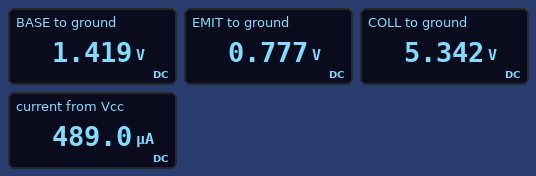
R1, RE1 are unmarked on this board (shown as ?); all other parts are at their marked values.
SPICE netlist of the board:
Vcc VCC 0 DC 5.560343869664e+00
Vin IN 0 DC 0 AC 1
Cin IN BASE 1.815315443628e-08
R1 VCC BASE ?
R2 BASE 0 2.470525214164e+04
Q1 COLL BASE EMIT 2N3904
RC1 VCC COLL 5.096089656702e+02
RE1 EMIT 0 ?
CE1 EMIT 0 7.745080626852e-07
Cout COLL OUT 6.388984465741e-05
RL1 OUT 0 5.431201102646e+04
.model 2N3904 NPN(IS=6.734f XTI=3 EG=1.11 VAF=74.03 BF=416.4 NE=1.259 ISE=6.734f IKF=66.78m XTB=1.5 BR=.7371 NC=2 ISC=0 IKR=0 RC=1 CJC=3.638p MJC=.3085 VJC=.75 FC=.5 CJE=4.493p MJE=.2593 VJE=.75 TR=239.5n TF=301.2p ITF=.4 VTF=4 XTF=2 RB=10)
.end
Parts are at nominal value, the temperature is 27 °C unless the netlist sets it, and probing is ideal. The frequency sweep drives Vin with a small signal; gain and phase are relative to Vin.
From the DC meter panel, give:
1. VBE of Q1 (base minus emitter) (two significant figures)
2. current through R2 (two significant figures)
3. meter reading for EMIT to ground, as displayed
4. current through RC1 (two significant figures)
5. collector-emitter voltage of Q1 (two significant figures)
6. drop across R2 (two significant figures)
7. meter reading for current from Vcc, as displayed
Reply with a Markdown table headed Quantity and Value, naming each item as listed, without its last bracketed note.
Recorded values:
| Quantity | Value |
|---|---|
| VBE of Q1 (base minus emitter) | 640 mV |
| current through R2 | 57 µA |
| meter reading for EMIT to ground, as displayed | 0.777 V |
| current through RC1 | 430 µA |
| collector-emitter voltage of Q1 | 4.6 V |
| drop across R2 | 1.4 V |
| meter reading for current from Vcc, as displayed | 489.0 µA |
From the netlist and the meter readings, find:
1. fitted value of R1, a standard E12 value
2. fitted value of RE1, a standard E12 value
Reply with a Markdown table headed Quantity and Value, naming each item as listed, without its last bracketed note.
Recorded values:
| Quantity | Value |
|---|---|
| fitted value of R1, a standard E12 value | 68 kΩ |
| fitted value of RE1, a standard E12 value | 1.8 kΩ |
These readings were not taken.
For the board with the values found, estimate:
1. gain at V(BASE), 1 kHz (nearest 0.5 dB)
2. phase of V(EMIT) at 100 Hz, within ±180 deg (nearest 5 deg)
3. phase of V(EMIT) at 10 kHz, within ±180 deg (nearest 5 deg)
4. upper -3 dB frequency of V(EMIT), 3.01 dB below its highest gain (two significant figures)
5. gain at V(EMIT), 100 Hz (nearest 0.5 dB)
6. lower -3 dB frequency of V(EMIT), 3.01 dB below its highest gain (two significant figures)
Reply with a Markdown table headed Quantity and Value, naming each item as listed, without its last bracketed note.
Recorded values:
| Quantity | Value |
|---|---|
| gain at V(BASE), 1 kHz | -3.0 dB |
| phase of V(EMIT) at 100 Hz, within ±180 deg | 75 deg |
| phase of V(EMIT) at 10 kHz, within ±180 deg | -65 deg |
| upper -3 dB frequency of V(EMIT), 3.01 dB below its highest gain | 5.3 kHz |
| gain at V(EMIT), 100 Hz | -15.0 dB |
| lower -3 dB frequency of V(EMIT), 3.01 dB below its highest gain | 340 Hz |
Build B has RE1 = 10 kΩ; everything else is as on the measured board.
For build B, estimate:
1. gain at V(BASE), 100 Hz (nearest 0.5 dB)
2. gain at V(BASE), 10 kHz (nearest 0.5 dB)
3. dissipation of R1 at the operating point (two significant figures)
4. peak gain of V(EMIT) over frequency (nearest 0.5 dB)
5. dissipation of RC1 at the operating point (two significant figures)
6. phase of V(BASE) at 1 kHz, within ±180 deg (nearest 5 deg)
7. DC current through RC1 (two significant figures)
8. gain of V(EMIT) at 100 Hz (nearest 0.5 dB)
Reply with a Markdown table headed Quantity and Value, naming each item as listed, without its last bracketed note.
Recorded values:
| Quantity | Value |
|---|---|
| gain at V(BASE), 100 Hz | -14.0 dB |
| gain at V(BASE), 10 kHz | 0 dB |
| dissipation of R1 at the operating point | 250 µW |
| peak gain of V(EMIT) over frequency | -6.5 dB |
| dissipation of RC1 at the operating point | 3.7 µW |
| phase of V(BASE) at 1 kHz, within ±180 deg | 30 deg |
| DC current through RC1 | 86 µA |
| gain of V(EMIT) at 100 Hz | -14.5 dB |
